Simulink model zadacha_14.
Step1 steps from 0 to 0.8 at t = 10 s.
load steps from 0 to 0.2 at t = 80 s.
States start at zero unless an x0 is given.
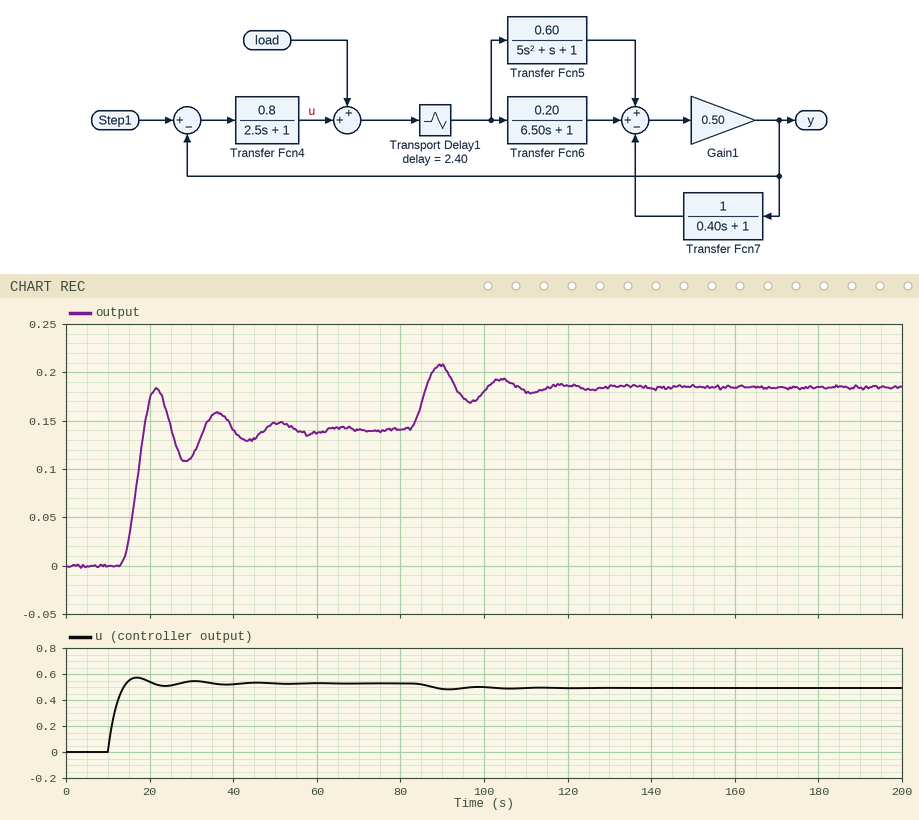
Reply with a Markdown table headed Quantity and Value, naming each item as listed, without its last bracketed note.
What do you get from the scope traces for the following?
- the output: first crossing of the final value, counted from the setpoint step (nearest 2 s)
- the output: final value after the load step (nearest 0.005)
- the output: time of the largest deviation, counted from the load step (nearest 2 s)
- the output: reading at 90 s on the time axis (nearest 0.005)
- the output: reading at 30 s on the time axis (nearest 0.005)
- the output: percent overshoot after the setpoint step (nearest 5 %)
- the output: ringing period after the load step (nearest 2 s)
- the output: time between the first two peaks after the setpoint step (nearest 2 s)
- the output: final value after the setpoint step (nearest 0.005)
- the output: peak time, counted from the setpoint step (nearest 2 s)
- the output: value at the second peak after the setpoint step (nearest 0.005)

| Quantity | Value |
|---|---|
| the output: first crossing of the final value, counted from the setpoint step | 8 s |
| the output: final value after the load step | 0.185 |
| the output: time of the largest deviation, counted from the load step | 10 s |
| the output: reading at 90 s on the time axis | 0.205 |
| the output: reading at 30 s on the time axis | 0.110 |
| the output: percent overshoot after the setpoint step | 30 % |
| the output: ringing period after the load step | 14 s |
| the output: time between the first two peaks after the setpoint step | 14 s |
| the output: final value after the setpoint step | 0.140 |
| the output: peak time, counted from the setpoint step | 12 s |
| the output: value at the second peak after the setpoint step | 0.160 |
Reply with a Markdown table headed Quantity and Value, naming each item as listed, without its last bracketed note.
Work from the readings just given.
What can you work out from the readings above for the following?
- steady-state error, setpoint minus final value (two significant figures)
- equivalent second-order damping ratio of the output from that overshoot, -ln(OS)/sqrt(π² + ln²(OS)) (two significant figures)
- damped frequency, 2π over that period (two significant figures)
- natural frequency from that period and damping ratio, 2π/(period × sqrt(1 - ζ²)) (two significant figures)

| Quantity | Value |
|---|---|
| steady-state error, setpoint minus final value | 0.66 |
| equivalent second-order damping ratio of the output from that overshoot, -ln(OS)/sqrt(π² + ln²(OS)) | 0.36 |
| damped frequency, 2π over that period | 0.45 rad/s |
| natural frequency from that period and damping ratio, 2π/(period × sqrt(1 - ζ²)) | 0.48 rad/s |
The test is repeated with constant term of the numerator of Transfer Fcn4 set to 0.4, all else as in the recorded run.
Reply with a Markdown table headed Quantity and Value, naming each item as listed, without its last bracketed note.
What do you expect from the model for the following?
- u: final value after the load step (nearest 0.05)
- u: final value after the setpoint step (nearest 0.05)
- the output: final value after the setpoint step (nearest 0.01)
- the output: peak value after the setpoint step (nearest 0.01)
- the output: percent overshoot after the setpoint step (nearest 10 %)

| Quantity | Value |
|---|---|
| u: final value after the load step | 0.25 |
| u: final value after the setpoint step | 0.30 |
| the output: final value after the setpoint step | 0.08 |
| the output: peak value after the setpoint step | 0.09 |
| the output: percent overshoot after the setpoint step | 20 % |
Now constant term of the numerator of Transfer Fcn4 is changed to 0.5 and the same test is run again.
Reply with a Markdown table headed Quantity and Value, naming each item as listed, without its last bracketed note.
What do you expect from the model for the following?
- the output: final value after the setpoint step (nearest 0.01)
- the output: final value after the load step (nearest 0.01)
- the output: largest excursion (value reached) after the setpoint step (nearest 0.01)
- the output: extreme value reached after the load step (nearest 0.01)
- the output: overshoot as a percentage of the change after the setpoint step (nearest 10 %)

| Quantity | Value |
|---|---|
| the output: final value after the setpoint step | 0.09 |
| the output: final value after the load step | 0.14 |
| the output: largest excursion (value reached) after the setpoint step | 0.12 |
| the output: extreme value reached after the load step | 0.16 |
| the output: overshoot as a percentage of the change after the setpoint step | 20 % |
